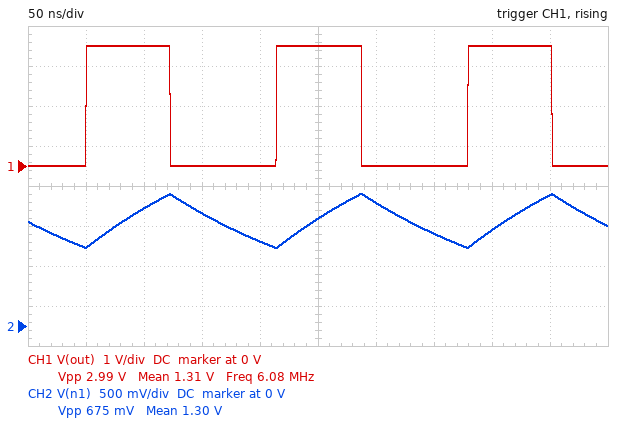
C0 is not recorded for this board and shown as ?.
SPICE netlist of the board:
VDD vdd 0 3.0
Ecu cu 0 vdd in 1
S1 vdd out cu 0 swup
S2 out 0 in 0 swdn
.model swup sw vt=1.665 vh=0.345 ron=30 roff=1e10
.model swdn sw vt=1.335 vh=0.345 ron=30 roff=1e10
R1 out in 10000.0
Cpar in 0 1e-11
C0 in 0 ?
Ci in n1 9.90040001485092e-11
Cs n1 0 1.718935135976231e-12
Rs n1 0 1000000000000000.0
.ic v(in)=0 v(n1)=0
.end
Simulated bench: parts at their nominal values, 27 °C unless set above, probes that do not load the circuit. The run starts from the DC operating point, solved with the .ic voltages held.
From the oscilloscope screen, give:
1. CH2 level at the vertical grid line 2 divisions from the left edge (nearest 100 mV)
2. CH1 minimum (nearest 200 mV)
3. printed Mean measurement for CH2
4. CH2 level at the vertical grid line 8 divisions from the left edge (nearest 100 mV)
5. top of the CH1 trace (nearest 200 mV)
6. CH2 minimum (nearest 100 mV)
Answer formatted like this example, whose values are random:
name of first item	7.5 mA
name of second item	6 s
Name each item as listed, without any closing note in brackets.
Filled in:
CH2 level at the vertical grid line 2 divisions from the left edge	1.5 V
CH1 minimum	0 V
printed Mean measurement for CH2	1.30 V
CH2 level at the vertical grid line 8 divisions from the left edge	1.2 V
top of the CH1 trace	3.0 V
CH2 minimum	1.0 V
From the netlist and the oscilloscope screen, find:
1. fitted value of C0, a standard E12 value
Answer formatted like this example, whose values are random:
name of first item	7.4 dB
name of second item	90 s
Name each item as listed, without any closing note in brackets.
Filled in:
fitted value of C0, a standard E12 value	5.6 pF
